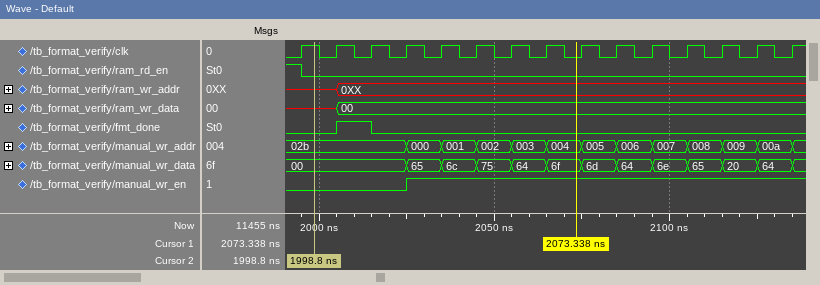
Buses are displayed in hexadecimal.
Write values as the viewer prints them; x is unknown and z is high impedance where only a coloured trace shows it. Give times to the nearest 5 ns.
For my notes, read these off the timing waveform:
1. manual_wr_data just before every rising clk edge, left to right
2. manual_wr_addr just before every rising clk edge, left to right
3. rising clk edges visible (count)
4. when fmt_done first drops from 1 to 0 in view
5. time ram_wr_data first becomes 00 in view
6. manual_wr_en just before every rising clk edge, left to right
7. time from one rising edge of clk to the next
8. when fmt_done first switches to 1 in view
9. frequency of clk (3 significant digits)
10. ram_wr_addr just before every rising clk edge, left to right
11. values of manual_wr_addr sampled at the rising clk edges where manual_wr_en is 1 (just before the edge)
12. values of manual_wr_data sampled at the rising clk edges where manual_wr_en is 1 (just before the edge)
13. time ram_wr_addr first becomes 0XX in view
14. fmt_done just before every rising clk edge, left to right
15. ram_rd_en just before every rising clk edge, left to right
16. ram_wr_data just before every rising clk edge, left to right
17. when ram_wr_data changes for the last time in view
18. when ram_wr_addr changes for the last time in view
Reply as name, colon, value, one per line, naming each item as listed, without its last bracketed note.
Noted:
manual_wr_data just before every rising clk edge, left to right: 00, 00, 00, 00, 65, 6c, 75, 64, 6f, 6d, 64, 6e, 65, 20, 64
manual_wr_addr just before every rising clk edge, left to right: 02b, 02b, 02b, 02b, 000, 001, 002, 003, 004, 005, 006, 007, 008, 009, 00a
rising clk edges visible: 15
when fmt_done first drops from 1 to 0 in view: 2015 ns
time ram_wr_data first becomes 00 in view: 2005 ns
manual_wr_en just before every rising clk edge, left to right: 0 0 0 0 1 1 1 1 1 1 1 1 1 1 1
time from one rising edge of clk to the next: 10 ns
when fmt_done first switches to 1 in view: 2005 ns
frequency of clk: 100 MHz
ram_wr_addr just before every rising clk edge, left to right: x, x, 0XX, 0XX, 0XX, 0XX, 0XX, 0XX, 0XX, 0XX, 0XX, 0XX, 0XX, 0XX, 0XX
values of manual_wr_addr sampled at the rising clk edges where manual_wr_en is 1: 000, 001, 002, 003, 004, 005, 006, 007, 008, 009, 00a
values of manual_wr_data sampled at the rising clk edges where manual_wr_en is 1: 65, 6c, 75, 64, 6f, 6d, 64, 6e, 65, 20, 64
time ram_wr_addr first becomes 0XX in view: 2005 ns
fmt_done just before every rising clk edge, left to right: 0 0 1 0 0 0 0 0 0 0 0 0 0 0 0
ram_rd_en just before every rising clk edge, left to right: 1 0 0 0 0 0 0 0 0 0 0 0 0 0 0
ram_wr_data just before every rising clk edge, left to right: x, x, 00, 00, 00, 00, 00, 00, 00, 00, 00, 00, 00, 00, 00
when ram_wr_data changes for the last time in view: 2005 ns
when ram_wr_addr changes for the last time in view: 2005 ns
